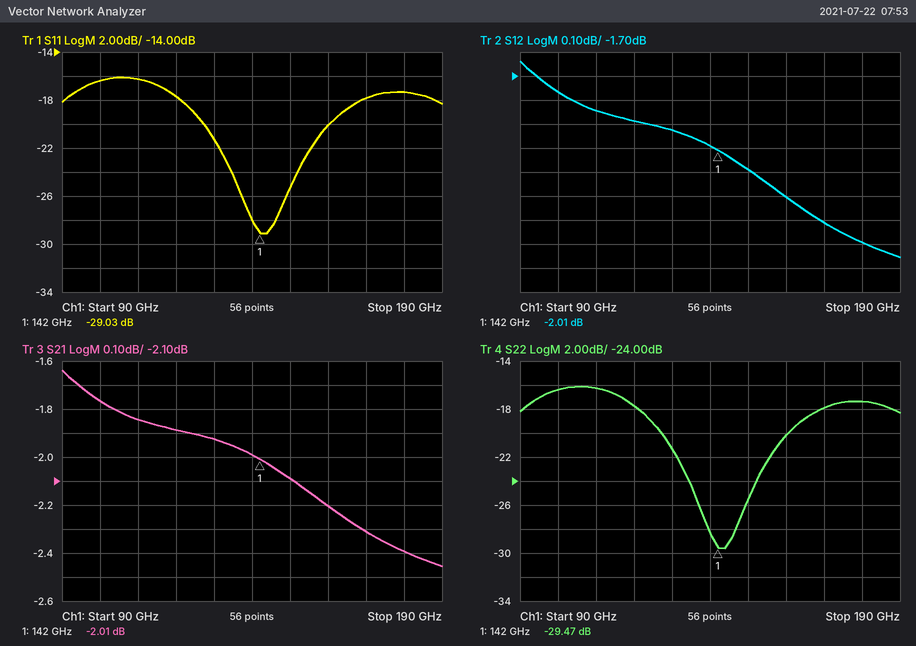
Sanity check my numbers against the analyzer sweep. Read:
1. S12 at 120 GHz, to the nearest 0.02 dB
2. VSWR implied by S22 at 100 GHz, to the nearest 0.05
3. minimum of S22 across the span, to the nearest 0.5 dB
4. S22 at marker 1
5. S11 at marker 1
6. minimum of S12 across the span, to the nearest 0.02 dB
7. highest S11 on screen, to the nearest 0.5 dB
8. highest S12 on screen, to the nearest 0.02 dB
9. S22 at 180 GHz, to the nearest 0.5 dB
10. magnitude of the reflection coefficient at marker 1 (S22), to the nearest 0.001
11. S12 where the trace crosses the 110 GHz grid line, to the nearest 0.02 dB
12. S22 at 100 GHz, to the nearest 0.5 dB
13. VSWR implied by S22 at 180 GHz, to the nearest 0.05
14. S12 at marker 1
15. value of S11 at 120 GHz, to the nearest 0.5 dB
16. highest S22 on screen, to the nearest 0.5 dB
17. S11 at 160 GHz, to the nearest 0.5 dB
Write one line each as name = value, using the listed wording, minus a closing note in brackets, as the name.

S12 at 120 GHz, to the nearest 0.02 dB = -1.88 dB
VSWR implied by S22 at 100 GHz, to the nearest 0.05 = 1.35
minimum of S22 across the span, to the nearest 0.5 dB = -29.5 dB
S22 at marker 1 = -29.47 dB
S11 at marker 1 = -29.03 dB
minimum of S12 across the span, to the nearest 0.02 dB = -2.46 dB
highest S11 on screen, to the nearest 0.5 dB = -16.0 dB
highest S12 on screen, to the nearest 0.02 dB = -1.64 dB
S22 at 180 GHz, to the nearest 0.5 dB = -17.5 dB
magnitude of the reflection coefficient at marker 1 (S22), to the nearest 0.001 = 0.034
S12 where the trace crosses the 110 GHz grid line, to the nearest 0.02 dB = -1.84 dB
S22 at 100 GHz, to the nearest 0.5 dB = -16.5 dB
VSWR implied by S22 at 180 GHz, to the nearest 0.05 = 1.30
S12 at marker 1 = -2.01 dB
value of S11 at 120 GHz, to the nearest 0.5 dB = -17.5 dB
highest S22 on screen, to the nearest 0.5 dB = -16.0 dB
S11 at 160 GHz, to the nearest 0.5 dB = -20.0 dB
